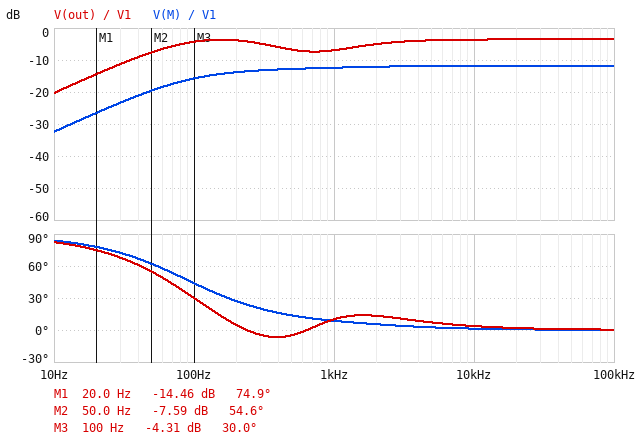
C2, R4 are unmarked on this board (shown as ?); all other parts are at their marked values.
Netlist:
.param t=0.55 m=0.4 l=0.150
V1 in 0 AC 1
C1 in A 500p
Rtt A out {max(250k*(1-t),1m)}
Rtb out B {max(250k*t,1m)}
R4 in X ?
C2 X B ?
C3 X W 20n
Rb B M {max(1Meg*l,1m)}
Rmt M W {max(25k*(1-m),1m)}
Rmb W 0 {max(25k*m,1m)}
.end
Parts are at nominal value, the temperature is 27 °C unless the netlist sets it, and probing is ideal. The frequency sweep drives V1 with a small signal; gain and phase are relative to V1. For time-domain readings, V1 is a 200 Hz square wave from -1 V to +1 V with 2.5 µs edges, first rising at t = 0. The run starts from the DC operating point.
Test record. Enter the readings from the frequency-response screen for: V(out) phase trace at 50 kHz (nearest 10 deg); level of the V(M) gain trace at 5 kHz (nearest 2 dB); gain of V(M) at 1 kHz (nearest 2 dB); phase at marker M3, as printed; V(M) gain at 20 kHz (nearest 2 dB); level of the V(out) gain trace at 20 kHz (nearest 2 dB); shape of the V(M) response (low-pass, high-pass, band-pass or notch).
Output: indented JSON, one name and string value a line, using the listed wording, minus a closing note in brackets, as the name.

{
  "V(out) phase trace at 50 kHz": "0 deg",
  "level of the V(M) gain trace at 5 kHz": "-12 dB",
  "gain of V(M) at 1 kHz": "-12 dB",
  "phase at marker M3, as printed": "30.0 deg",
  "V(M) gain at 20 kHz": "-12 dB",
  "level of the V(out) gain trace at 20 kHz": "-4 dB",
  "shape of the V(M) response": "high-pass"
}
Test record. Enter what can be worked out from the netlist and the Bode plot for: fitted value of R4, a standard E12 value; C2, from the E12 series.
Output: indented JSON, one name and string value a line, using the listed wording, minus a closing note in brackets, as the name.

{
  "fitted value of R4, a standard E12 value": "33 kΩ",
  "C2, from the E12 series": "6.8 nF"
}
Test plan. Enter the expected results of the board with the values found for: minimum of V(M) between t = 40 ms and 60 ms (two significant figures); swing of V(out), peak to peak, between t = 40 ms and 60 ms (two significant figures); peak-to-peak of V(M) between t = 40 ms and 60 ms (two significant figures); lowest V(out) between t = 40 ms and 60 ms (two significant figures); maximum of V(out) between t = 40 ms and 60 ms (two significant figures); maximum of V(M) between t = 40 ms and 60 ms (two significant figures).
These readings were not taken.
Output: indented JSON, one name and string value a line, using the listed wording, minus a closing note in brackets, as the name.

{
  "minimum of V(M) between t = 40 ms and 60 ms": "-430 mV",
  "swing of V(out), peak to peak, between t = 40 ms and 60 ms": "1.8 V",
  "peak-to-peak of V(M) between t = 40 ms and 60 ms": "860 mV",
  "lowest V(out) between t = 40 ms and 60 ms": "-900 mV",
  "maximum of V(out) between t = 40 ms and 60 ms": "900 mV",
  "maximum of V(M) between t = 40 ms and 60 ms": "430 mV"
}
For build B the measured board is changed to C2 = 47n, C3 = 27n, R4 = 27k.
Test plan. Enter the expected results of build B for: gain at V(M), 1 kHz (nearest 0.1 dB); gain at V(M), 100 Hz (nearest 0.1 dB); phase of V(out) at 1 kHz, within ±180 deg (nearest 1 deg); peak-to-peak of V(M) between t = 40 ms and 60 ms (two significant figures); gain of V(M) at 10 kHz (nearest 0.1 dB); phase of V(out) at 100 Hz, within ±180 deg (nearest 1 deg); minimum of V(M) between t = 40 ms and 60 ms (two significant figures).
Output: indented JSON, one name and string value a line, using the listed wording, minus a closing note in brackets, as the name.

{
  "gain at V(M), 1 kHz": "-11.3 dB",
  "gain at V(M), 100 Hz": "-15.0 dB",
  "phase of V(out) at 1 kHz, within ±180 deg": "13 deg",
  "peak-to-peak of V(M) between t = 40 ms and 60 ms": "900 mV",
  "gain of V(M) at 10 kHz": "-10.7 dB",
  "phase of V(out) at 100 Hz, within ±180 deg": "-8 deg",
  "minimum of V(M) between t = 40 ms and 60 ms": "-450 mV"
}
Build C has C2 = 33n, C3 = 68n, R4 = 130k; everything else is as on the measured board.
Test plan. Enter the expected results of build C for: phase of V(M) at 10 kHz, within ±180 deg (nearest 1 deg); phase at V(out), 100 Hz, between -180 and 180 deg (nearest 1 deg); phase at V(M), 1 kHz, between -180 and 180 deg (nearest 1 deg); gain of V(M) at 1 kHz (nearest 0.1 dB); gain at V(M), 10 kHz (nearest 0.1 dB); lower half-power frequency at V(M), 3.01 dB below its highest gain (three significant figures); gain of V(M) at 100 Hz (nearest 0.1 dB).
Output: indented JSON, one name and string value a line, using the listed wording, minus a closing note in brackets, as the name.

{
  "phase of V(M) at 10 kHz, within ±180 deg": "2 deg",
  "phase at V(out), 100 Hz, between -180 and 180 deg": "-23 deg",
  "phase at V(M), 1 kHz, between -180 and 180 deg": "10 deg",
  "gain of V(M) at 1 kHz": "-21.3 dB",
  "gain at V(M), 10 kHz": "-19.6 dB",
  "lower half-power frequency at V(M), 3.01 dB below its highest gain": "13.5 Hz",
  "gain of V(M) at 100 Hz": "-22.3 dB"
}
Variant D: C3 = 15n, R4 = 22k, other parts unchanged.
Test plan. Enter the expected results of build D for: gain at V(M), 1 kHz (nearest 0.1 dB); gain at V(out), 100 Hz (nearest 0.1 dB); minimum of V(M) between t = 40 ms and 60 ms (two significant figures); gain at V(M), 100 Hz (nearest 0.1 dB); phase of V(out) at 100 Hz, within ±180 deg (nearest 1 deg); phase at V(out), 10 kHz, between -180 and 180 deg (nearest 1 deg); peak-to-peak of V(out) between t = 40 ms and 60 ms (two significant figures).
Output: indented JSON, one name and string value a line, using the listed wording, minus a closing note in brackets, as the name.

{
  "gain at V(M), 1 kHz": "-10.3 dB",
  "gain at V(out), 100 Hz": "-3.6 dB",
  "minimum of V(M) between t = 40 ms and 60 ms": "-600 mV",
  "gain at V(M), 100 Hz": "-16.2 dB",
  "phase of V(out) at 100 Hz, within ±180 deg": "38 deg",
  "phase at V(out), 10 kHz, between -180 and 180 deg": "3 deg",
  "peak-to-peak of V(out) between t = 40 ms and 60 ms": "2.0 V"
}
